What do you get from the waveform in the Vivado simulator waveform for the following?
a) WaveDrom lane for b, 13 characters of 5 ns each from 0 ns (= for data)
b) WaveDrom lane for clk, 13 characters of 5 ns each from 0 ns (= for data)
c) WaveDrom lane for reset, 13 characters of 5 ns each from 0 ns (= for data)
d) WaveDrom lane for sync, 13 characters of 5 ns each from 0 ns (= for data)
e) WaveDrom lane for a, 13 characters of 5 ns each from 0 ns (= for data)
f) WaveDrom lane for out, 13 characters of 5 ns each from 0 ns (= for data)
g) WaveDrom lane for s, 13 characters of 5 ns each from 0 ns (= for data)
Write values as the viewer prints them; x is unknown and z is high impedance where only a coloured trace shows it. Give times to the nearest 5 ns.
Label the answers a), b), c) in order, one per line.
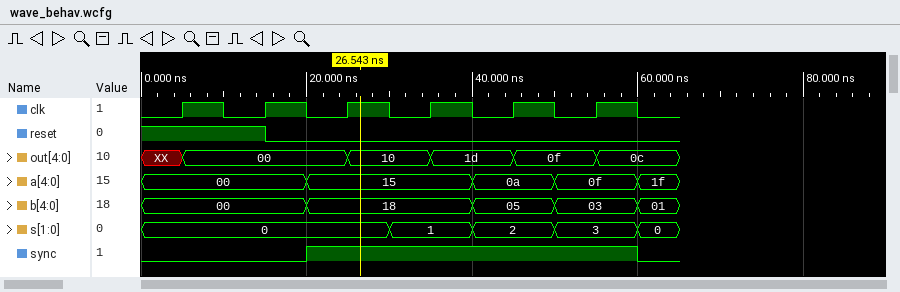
a) {name: 'b', wave: '=...=...=.=.=', data: '00 18 05 03 01'}
b) {name: 'clk', wave: '0101010101010'}
c) {name: 'reset', wave: '1..0.........'}
d) {name: 'sync', wave: '0...1.......0'}
e) {name: 'a', wave: '=...=...=.=.=', data: '00 15 0a 0f 1f'}
f) {name: 'out', wave: 'x=...=.=.=.=.', data: '00 10 1d 0f 0c'}
g) {name: 's', wave: '=.....=.=.=.=', data: '0 1 2 3 0'}
